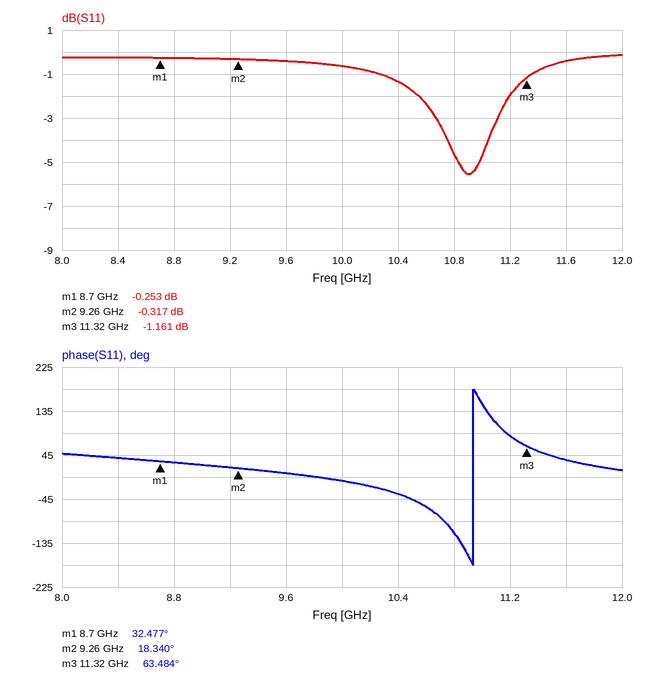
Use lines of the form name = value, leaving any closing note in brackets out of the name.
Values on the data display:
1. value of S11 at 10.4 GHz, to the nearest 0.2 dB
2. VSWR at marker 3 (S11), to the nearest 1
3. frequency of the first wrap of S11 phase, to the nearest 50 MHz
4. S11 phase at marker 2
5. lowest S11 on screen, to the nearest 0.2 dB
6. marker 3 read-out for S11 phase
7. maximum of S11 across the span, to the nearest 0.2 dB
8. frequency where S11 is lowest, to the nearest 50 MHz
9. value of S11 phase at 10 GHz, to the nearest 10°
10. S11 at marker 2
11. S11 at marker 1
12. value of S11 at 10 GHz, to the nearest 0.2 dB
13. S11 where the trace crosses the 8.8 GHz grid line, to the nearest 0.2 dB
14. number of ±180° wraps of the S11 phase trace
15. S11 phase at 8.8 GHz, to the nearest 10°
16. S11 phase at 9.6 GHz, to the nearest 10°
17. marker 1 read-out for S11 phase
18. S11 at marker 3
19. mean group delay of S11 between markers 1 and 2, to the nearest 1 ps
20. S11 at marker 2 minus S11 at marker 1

value of S11 at 10.4 GHz, to the nearest 0.2 dB = -1.4 dB
VSWR at marker 3 (S11), to the nearest 1 = 15
frequency of the first wrap of S11 phase, to the nearest 50 MHz = 10.95 GHz
S11 phase at marker 2 = 18.340°
lowest S11 on screen, to the nearest 0.2 dB = -5.6 dB
marker 3 read-out for S11 phase = 63.484°
maximum of S11 across the span, to the nearest 0.2 dB = -0.2 dB
frequency where S11 is lowest, to the nearest 50 MHz = 10.90 GHz
value of S11 phase at 10 GHz, to the nearest 10° = -10°
S11 at marker 2 = -0.317 dB
S11 at marker 1 = -0.253 dB
value of S11 at 10 GHz, to the nearest 0.2 dB = -0.6 dB
S11 where the trace crosses the 8.8 GHz grid line, to the nearest 0.2 dB = -0.2 dB
number of ±180° wraps of the S11 phase trace = 1
S11 phase at 8.8 GHz, to the nearest 10° = 30°
S11 phase at 9.6 GHz, to the nearest 10° = 10°
marker 1 read-out for S11 phase = 32.477°
S11 at marker 3 = -1.161 dB
mean group delay of S11 between markers 1 and 2, to the nearest 1 ps = 70 ps
S11 at marker 2 minus S11 at marker 1 = -0.064 dB
